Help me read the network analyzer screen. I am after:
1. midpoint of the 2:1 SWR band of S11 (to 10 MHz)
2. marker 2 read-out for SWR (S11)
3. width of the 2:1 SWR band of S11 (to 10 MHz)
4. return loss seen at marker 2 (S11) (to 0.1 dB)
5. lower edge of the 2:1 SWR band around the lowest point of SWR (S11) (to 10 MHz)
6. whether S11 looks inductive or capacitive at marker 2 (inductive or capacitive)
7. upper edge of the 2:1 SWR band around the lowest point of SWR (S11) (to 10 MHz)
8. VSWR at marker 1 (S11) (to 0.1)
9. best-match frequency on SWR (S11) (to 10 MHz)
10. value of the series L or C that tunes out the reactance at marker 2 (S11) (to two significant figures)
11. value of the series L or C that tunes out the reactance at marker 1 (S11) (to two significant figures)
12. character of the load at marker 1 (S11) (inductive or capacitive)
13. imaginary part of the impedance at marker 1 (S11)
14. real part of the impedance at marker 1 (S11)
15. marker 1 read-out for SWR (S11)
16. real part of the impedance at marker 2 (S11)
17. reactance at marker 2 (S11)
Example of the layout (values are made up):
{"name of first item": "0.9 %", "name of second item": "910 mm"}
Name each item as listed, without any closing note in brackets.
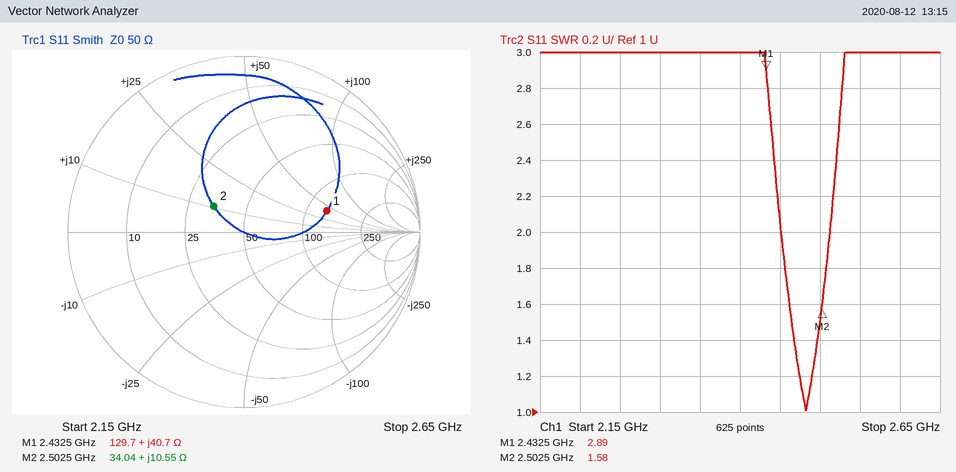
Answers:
{"midpoint of the 2:1 SWR band of S11": "2.48 GHz", "marker 2 read-out for SWR": "1.58", "width of the 2:1 SWR band of S11": "60 MHz", "return loss seen at marker 2 (S11)": "12.9 dB", "lower edge of the 2:1 SWR band around the lowest point of SWR (S11)": "2.45 GHz", "whether S11 looks inductive or capacitive at marker 2": "inductive", "upper edge of the 2:1 SWR band around the lowest point of SWR (S11)": "2.51 GHz", "VSWR at marker 1 (S11)": "2.9", "best-match frequency on SWR (S11)": "2.48 GHz", "value of the series L or C that tunes out the reactance at marker 2 (S11)": "6.0 pF", "value of the series L or C that tunes out the reactance at marker 1 (S11)": "1.6 pF", "character of the load at marker 1 (S11)": "inductive", "imaginary part of the impedance at marker 1": "+40.7 Ω", "real part of the impedance at marker 1": "129.7 Ω", "marker 1 read-out for SWR": "2.89", "real part of the impedance at marker 2": "34.04 Ω", "reactance at marker 2": "+10.55 Ω"}
